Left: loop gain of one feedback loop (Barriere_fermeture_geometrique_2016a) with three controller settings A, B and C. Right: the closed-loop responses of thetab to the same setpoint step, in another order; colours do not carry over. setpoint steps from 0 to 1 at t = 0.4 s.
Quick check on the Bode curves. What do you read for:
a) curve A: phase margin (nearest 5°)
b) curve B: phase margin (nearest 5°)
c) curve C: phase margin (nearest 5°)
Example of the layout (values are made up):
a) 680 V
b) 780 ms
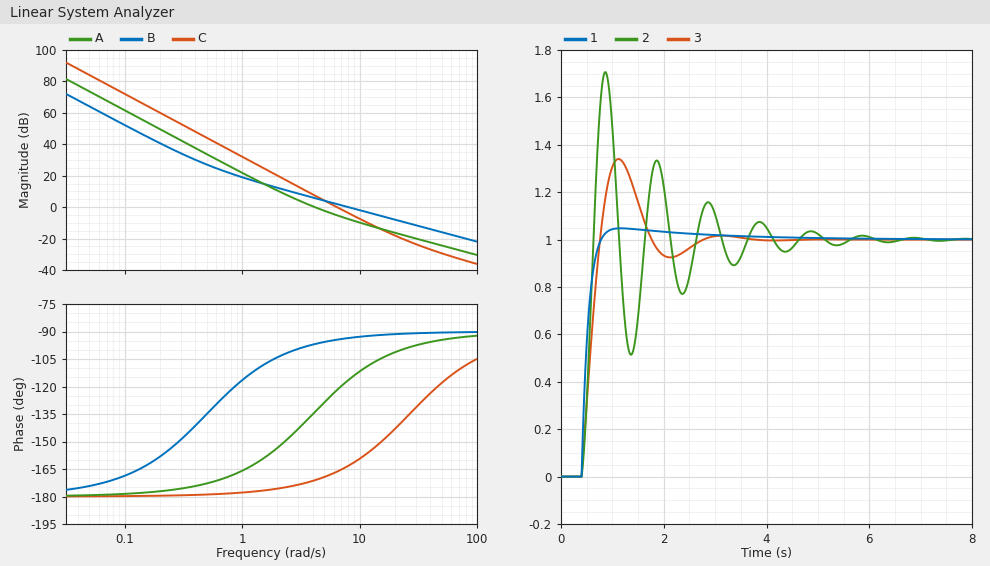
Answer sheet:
a) 45°
b) 85°
c) 15°
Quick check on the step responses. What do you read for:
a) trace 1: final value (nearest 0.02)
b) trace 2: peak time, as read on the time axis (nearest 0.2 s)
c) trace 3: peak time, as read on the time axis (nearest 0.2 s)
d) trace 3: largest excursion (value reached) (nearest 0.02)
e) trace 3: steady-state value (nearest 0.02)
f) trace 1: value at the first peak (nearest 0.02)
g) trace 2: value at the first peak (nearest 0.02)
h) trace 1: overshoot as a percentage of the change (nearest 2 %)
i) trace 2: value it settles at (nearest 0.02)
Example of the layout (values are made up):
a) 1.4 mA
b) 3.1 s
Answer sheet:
a) 1.00
b) 0.8 s
c) 1.2 s
d) 1.34
e) 1.00
f) 1.04
g) 1.70
h) 4 %
i) 1.00
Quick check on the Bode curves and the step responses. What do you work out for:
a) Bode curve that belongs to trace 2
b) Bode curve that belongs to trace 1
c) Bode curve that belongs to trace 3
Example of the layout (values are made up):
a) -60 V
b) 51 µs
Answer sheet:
a) C
b) B
c) A
